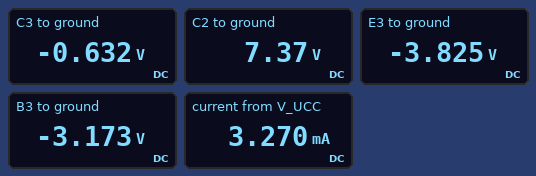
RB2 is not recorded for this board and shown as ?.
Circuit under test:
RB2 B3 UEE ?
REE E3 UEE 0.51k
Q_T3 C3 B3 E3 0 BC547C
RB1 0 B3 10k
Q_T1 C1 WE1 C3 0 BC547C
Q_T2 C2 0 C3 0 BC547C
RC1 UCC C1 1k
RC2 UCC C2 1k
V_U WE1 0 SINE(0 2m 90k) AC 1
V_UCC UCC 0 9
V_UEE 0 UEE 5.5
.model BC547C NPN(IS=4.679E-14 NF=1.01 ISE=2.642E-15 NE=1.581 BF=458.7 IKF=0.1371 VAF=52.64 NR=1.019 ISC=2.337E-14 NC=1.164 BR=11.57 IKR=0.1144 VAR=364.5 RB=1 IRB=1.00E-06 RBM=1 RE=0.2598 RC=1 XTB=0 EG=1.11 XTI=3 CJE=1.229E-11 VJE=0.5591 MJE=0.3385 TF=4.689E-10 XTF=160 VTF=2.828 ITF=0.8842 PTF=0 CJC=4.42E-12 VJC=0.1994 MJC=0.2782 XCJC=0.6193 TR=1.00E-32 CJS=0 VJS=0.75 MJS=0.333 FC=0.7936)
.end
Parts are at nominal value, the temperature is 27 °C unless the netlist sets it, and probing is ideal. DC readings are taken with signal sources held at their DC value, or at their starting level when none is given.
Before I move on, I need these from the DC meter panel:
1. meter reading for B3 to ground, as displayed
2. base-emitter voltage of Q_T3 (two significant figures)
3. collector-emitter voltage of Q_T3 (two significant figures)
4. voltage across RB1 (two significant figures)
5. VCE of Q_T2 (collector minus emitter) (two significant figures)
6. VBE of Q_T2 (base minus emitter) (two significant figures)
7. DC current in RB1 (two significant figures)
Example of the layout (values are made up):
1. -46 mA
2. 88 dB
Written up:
1. -3.173 V
2. 650 mV
3. 3.2 V
4. 3.2 V
5. 8.0 V
6. 630 mV
7. 320 µA
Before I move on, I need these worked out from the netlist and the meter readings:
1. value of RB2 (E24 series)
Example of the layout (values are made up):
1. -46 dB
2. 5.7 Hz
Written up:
1. 7.5 kΩ
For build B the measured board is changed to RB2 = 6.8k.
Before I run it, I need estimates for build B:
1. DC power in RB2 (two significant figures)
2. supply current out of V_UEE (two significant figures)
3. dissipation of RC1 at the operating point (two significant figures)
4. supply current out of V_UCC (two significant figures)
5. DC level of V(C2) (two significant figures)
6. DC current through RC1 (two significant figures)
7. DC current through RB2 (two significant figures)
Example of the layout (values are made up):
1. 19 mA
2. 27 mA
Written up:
1. 710 µW
2. 3.4 mA
3. 2.3 mW
4. 3.0 mA
5. 7.5 V
6. 1.5 mA
7. 320 µA
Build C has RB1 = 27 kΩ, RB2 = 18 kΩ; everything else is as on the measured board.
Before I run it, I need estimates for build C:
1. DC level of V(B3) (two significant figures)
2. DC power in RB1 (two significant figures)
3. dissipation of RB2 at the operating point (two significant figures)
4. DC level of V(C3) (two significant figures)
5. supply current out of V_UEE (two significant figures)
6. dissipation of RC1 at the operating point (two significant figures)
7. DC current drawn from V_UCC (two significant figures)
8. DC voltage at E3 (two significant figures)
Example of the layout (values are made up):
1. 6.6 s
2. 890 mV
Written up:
1. -3.4 V
2. 420 µW
3. 250 µW
4. -630 mV
5. 3.0 mA
6. 2.1 mW
7. 2.9 mA
8. -4.0 V
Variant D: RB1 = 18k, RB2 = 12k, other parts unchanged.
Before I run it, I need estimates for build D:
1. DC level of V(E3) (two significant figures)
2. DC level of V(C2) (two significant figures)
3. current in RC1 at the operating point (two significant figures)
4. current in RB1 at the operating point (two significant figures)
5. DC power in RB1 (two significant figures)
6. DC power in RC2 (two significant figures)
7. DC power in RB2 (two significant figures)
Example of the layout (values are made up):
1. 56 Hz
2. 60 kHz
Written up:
1. -4.0 V
2. 7.5 V
3. 1.5 mA
4. 190 µA
5. 620 µW
6. 2.2 mW
7. 390 µW
